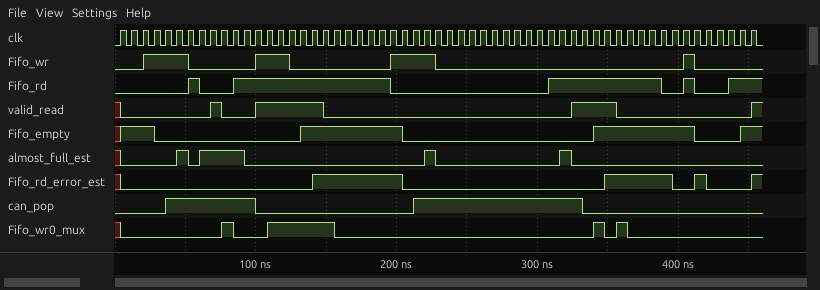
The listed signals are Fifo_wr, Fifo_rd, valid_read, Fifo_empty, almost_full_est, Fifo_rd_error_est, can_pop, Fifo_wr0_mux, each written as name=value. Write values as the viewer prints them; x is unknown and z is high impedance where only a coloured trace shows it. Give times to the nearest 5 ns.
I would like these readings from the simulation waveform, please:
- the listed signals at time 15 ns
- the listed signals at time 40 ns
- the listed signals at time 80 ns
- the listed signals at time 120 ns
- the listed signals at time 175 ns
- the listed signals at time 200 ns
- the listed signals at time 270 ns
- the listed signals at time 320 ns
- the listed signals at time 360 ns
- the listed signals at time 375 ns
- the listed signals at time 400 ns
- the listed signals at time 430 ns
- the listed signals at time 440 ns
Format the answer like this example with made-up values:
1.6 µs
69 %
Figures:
Fifo_wr=0, Fifo_rd=0, valid_read=0, Fifo_empty=1, almost_full_est=0, Fifo_rd_error_est=0, can_pop=0, Fifo_wr0_mux=0
Fifo_wr=1, Fifo_rd=0, valid_read=0, Fifo_empty=0, almost_full_est=0, Fifo_rd_error_est=0, can_pop=1, Fifo_wr0_mux=0
Fifo_wr=0, Fifo_rd=0, valid_read=0, Fifo_empty=0, almost_full_est=1, Fifo_rd_error_est=0, can_pop=1, Fifo_wr0_mux=1
Fifo_wr=1, Fifo_rd=1, valid_read=1, Fifo_empty=0, almost_full_est=0, Fifo_rd_error_est=0, can_pop=0, Fifo_wr0_mux=1
Fifo_wr=0, Fifo_rd=1, valid_read=0, Fifo_empty=1, almost_full_est=0, Fifo_rd_error_est=1, can_pop=0, Fifo_wr0_mux=0
Fifo_wr=1, Fifo_rd=0, valid_read=0, Fifo_empty=1, almost_full_est=0, Fifo_rd_error_est=1, can_pop=0, Fifo_wr0_mux=0
Fifo_wr=0, Fifo_rd=0, valid_read=0, Fifo_empty=0, almost_full_est=0, Fifo_rd_error_est=0, can_pop=1, Fifo_wr0_mux=0
Fifo_wr=0, Fifo_rd=1, valid_read=0, Fifo_empty=0, almost_full_est=1, Fifo_rd_error_est=0, can_pop=1, Fifo_wr0_mux=0
Fifo_wr=0, Fifo_rd=1, valid_read=0, Fifo_empty=1, almost_full_est=0, Fifo_rd_error_est=1, can_pop=0, Fifo_wr0_mux=1
Fifo_wr=0, Fifo_rd=1, valid_read=0, Fifo_empty=1, almost_full_est=0, Fifo_rd_error_est=1, can_pop=0, Fifo_wr0_mux=0
Fifo_wr=0, Fifo_rd=0, valid_read=0, Fifo_empty=1, almost_full_est=0, Fifo_rd_error_est=0, can_pop=0, Fifo_wr0_mux=0
Fifo_wr=0, Fifo_rd=0, valid_read=0, Fifo_empty=0, almost_full_est=0, Fifo_rd_error_est=0, can_pop=0, Fifo_wr0_mux=0
Fifo_wr=0, Fifo_rd=1, valid_read=0, Fifo_empty=0, almost_full_est=0, Fifo_rd_error_est=0, can_pop=0, Fifo_wr0_mux=0
